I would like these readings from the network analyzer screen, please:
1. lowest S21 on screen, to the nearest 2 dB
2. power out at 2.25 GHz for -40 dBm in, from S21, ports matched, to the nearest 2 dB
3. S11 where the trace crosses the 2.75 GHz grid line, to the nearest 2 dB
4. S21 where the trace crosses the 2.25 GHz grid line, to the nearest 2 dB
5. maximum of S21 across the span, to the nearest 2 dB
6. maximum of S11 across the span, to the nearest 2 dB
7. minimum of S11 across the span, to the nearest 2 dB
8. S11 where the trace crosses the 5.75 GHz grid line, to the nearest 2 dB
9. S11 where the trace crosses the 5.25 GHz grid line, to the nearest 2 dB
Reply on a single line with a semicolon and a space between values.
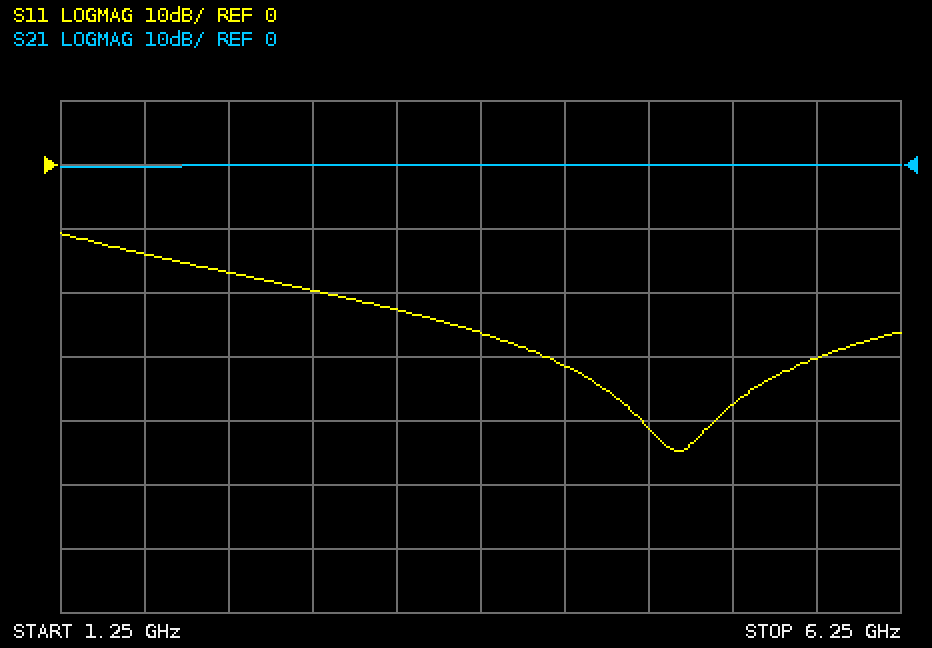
0 dB; -40 dBm; -20 dB; 0 dB; 0 dB; -10 dB; -44 dB; -30 dB; -38 dB
